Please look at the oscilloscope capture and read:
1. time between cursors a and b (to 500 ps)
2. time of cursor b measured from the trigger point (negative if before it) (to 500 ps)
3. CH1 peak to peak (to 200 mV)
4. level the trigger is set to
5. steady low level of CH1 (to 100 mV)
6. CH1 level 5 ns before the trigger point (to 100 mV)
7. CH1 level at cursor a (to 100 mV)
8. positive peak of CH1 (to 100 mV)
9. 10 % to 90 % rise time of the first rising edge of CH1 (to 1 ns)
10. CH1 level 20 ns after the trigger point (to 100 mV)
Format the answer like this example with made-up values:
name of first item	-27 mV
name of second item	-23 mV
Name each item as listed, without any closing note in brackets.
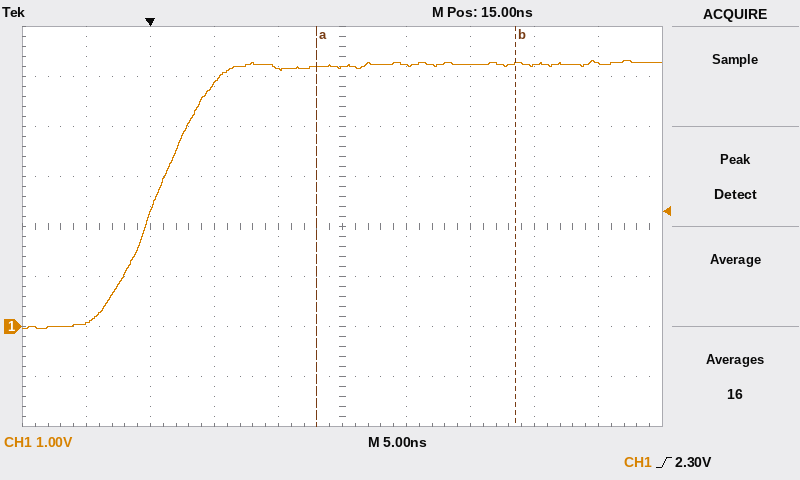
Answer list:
time between cursors a and b	15.5 ns
time of cursor b measured from the trigger point (negative if before it)	+28.5 ns
CH1 peak to peak	5.4 V
level the trigger is set to	2.30 V
steady low level of CH1	0.0 V
CH1 level 5 ns before the trigger point	100 mV
CH1 level at cursor a	5.2 V
positive peak of CH1	5.3 V
10 % to 90 % rise time of the first rising edge of CH1	8 ns
CH1 level 20 ns after the trigger point	5.2 V
